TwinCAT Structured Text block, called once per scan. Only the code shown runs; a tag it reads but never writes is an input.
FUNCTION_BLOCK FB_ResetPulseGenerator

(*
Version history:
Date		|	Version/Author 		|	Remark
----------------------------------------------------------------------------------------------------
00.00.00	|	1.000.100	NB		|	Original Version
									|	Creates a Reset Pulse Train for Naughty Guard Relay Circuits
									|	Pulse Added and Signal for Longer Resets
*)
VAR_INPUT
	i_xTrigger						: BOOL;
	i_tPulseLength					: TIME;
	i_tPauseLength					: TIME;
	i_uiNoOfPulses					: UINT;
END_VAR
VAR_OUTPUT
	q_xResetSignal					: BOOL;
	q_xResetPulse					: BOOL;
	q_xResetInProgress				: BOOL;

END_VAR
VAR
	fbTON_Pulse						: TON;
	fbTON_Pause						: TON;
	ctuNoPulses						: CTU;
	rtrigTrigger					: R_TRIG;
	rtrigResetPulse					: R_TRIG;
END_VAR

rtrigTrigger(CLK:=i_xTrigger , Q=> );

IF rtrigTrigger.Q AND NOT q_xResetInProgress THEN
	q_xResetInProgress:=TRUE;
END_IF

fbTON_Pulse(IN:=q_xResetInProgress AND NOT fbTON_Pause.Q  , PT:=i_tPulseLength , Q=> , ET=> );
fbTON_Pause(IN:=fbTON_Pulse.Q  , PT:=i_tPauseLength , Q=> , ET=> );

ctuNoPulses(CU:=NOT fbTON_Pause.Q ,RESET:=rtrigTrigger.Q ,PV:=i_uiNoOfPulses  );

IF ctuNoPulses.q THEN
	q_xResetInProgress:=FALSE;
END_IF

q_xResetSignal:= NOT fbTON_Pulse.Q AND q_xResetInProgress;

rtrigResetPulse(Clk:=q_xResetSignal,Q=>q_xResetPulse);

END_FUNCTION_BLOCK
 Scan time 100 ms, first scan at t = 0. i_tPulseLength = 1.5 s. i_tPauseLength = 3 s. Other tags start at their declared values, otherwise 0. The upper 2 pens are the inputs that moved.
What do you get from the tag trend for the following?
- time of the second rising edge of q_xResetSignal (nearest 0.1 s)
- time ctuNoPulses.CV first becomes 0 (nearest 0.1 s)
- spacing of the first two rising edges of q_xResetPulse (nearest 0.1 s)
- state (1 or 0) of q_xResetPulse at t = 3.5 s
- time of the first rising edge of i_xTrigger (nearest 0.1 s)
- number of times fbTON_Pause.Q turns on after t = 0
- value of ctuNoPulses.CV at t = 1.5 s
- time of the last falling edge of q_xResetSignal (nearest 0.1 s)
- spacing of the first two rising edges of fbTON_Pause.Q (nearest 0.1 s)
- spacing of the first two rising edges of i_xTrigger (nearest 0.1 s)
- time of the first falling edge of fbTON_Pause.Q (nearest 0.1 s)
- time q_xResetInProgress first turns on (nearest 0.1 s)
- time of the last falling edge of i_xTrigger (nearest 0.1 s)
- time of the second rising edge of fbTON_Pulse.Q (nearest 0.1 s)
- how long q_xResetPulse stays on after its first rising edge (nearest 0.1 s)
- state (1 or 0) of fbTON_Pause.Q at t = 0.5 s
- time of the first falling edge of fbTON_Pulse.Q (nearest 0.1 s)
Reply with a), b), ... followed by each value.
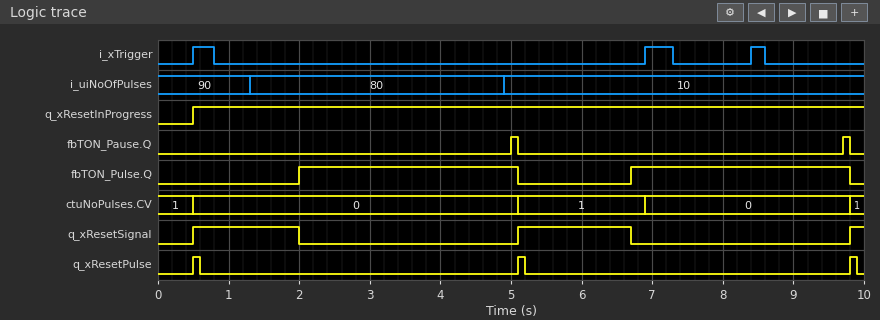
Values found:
a) 5.1 s
b) 0.5 s
c) 4.6 s
d) 0
e) 0.5 s
f) 2
g) 0
h) 6.7 s
i) 4.7 s
j) 6.4 s
k) 5.1 s
l) 0.5 s
m) 8.6 s
n) 6.7 s
o) 0.1 s
p) 0
q) 5.1 s
